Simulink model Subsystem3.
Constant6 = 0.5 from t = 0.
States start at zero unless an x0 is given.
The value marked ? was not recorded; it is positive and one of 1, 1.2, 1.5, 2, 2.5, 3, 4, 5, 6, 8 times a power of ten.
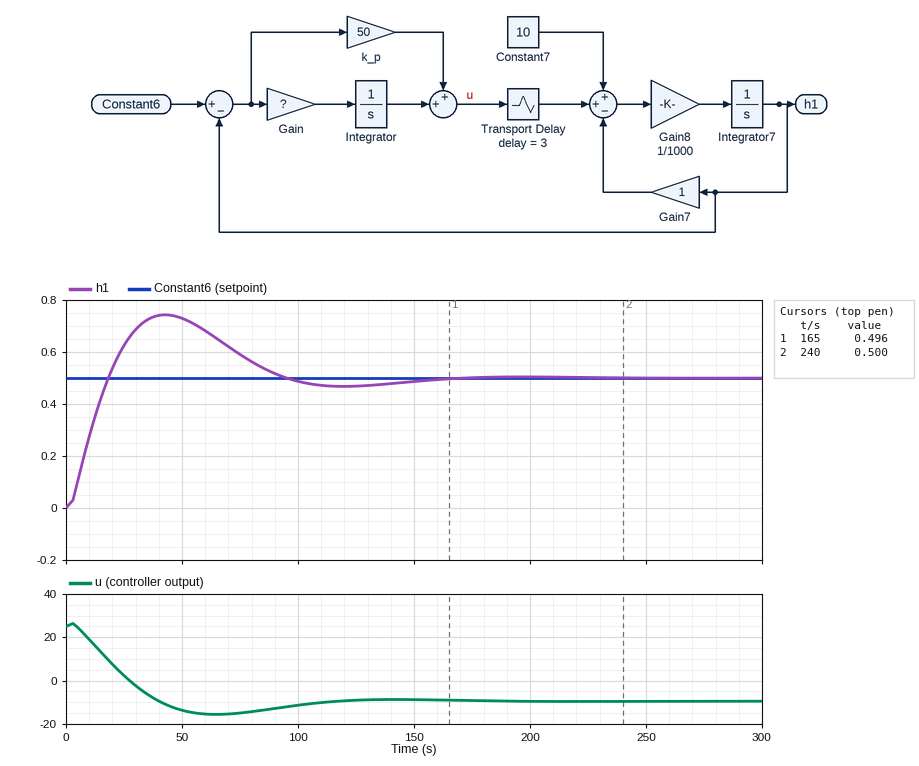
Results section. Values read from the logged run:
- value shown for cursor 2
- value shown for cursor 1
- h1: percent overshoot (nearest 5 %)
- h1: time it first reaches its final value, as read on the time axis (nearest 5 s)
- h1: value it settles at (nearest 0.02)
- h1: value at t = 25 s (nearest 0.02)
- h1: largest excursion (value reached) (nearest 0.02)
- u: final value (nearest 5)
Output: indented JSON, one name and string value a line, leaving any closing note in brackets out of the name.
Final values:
{
  "value shown for cursor 2": "0.500",
  "value shown for cursor 1": "0.496",
  "h1: percent overshoot": "50 %",
  "h1: time it first reaches its final value, as read on the time axis": "20 s",
  "h1: value it settles at": "0.50",
  "h1: value at t = 25 s": "0.62",
  "h1: largest excursion (value reached)": "0.74",
  "u: final value": "-10"
}
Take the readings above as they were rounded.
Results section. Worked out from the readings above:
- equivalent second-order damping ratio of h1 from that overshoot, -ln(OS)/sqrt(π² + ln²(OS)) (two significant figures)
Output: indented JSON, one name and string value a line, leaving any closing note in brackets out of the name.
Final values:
{
  "equivalent second-order damping ratio of h1 from that overshoot, -ln(OS)/sqrt(π² + ln²(OS))": "0.22"
}
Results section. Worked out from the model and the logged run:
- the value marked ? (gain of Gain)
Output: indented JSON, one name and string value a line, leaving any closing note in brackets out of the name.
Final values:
{
  "the value marked ?": "2"
}
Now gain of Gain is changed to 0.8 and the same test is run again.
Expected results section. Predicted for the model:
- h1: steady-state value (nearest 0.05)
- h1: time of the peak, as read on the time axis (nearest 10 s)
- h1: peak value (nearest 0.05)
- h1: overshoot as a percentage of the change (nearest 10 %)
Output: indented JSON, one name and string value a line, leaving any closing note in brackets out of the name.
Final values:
{
  "h1: steady-state value": "0.50",
  "h1: time of the peak, as read on the time axis": "50 s",
  "h1: peak value": "0.70",
  "h1: overshoot as a percentage of the change": "40 %"
}
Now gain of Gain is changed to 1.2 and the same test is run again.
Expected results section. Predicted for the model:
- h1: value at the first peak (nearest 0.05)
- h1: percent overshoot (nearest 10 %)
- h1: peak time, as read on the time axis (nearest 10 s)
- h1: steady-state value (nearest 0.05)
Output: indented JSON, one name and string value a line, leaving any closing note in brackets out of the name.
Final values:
{
  "h1: value at the first peak": "0.70",
  "h1: percent overshoot": "40 %",
  "h1: peak time, as read on the time axis": "50 s",
  "h1: steady-state value": "0.50"
}
